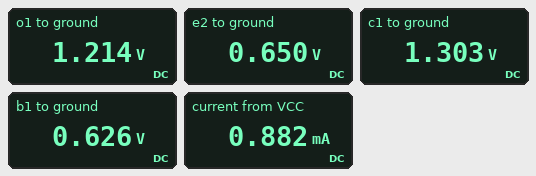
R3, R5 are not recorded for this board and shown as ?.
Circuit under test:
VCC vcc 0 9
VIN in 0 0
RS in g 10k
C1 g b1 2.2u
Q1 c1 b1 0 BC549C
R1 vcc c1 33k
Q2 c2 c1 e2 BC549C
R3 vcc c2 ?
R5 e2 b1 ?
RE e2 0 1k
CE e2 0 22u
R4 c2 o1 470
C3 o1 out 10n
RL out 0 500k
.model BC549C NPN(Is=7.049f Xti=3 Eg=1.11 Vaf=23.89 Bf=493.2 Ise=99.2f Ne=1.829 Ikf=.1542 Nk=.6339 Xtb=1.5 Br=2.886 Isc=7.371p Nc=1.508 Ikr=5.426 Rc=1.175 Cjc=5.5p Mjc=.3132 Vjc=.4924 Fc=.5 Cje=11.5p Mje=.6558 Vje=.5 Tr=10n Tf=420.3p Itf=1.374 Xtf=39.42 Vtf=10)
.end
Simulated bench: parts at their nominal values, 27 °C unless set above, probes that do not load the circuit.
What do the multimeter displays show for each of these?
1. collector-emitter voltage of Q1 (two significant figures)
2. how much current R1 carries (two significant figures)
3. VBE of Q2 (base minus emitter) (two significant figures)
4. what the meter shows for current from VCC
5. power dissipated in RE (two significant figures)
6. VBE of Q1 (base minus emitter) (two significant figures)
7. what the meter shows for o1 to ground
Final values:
1.3 V
230 µA
650 mV
0.882 mA
420 µW
630 mV
1.214 V
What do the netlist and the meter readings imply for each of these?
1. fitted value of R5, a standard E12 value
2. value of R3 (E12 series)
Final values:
47 kΩ
12 kΩ
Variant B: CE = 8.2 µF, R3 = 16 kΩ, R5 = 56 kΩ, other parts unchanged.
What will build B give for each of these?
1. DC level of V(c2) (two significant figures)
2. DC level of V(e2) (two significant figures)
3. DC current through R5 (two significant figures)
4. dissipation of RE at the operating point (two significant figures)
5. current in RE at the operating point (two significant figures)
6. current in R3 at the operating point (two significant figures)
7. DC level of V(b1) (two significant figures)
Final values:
670 mV
630 mV
290 nA
390 µW
630 µA
520 µA
610 mV
